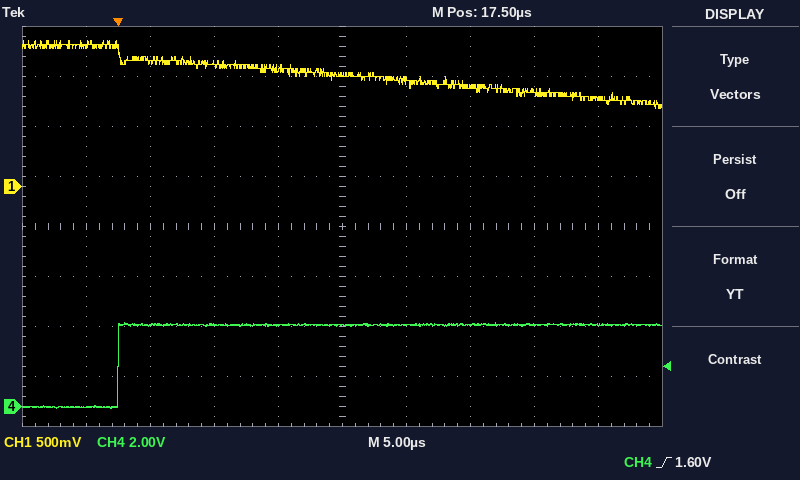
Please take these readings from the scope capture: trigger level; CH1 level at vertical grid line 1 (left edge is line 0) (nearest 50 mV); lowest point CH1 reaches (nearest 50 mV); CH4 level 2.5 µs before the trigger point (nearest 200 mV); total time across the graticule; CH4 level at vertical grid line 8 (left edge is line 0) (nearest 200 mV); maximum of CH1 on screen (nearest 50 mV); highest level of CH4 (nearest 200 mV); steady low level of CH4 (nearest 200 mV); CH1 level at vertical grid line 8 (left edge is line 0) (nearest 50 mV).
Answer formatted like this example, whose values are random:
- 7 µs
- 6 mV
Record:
- 1.60 V
- 1.40 V
- 800 mV
- 0.0 V
- 50 µs
- 3.2 V
- 1.45 V
- 3.4 V
- 0.0 V
- 950 mV
